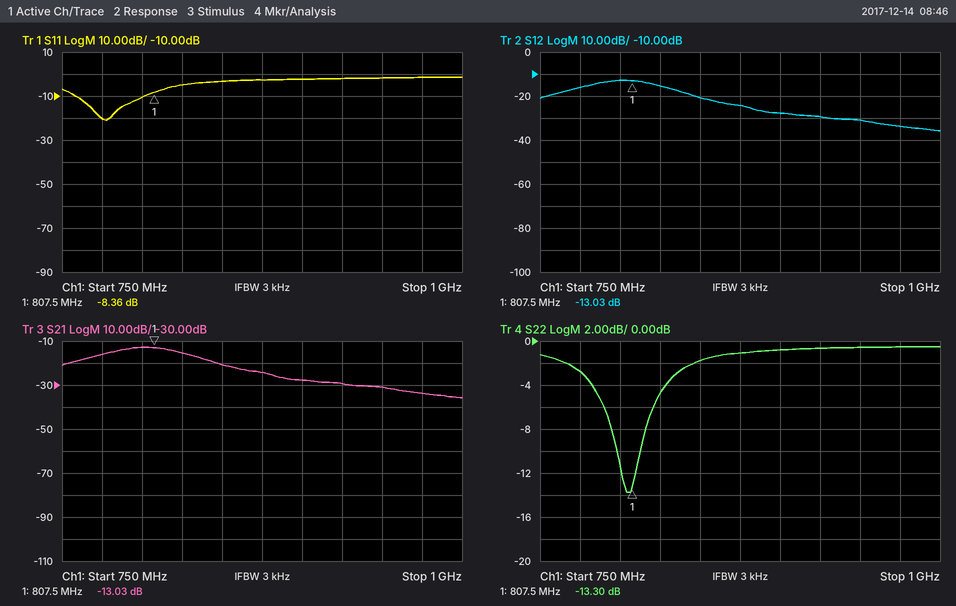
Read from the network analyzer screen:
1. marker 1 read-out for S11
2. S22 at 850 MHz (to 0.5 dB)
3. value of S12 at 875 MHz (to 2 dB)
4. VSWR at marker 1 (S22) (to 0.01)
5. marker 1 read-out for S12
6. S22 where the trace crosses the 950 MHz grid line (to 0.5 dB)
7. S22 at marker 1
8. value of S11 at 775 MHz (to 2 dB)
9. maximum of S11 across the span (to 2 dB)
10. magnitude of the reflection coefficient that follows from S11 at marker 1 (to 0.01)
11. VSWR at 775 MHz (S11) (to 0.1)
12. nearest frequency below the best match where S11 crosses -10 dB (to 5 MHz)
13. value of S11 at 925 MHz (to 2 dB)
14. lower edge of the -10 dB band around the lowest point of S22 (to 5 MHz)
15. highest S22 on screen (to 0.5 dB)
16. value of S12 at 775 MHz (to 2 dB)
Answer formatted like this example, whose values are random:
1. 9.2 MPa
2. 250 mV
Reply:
1. -8.36 dB
2. -2.0 dB
3. -24 dB
4. 1.55
5. -13.03 dB
6. -0.5 dB
7. -13.30 dB
8. -20 dB
9. -2 dB
10. 0.38
11. 1.2
12. 760 MHz
13. -2 dB
14. 800 MHz
15. -0.5 dB
16. -16 dB
